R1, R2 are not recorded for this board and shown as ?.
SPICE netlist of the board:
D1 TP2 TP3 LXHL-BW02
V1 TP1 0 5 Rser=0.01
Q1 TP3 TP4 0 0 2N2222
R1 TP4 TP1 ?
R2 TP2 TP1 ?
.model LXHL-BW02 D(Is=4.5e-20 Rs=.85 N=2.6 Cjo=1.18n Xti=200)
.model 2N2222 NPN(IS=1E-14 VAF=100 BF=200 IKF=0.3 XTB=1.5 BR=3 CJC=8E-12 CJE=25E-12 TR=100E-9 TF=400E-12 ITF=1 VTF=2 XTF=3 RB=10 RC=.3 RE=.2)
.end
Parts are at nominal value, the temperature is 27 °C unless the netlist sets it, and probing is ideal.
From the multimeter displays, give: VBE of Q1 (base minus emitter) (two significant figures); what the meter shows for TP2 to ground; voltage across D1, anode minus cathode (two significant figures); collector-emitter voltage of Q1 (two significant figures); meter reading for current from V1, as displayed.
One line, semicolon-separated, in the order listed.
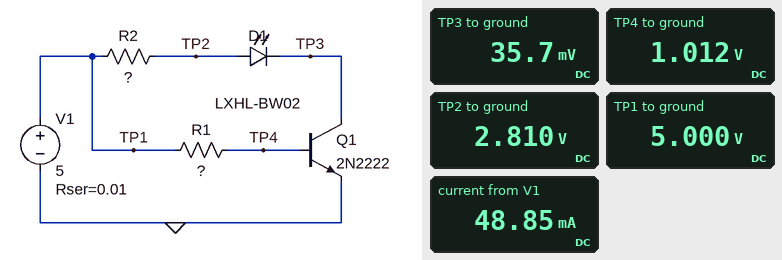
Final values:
1.0 V; 2.810 V; 2.8 V; 36 mV; 48.85 mA
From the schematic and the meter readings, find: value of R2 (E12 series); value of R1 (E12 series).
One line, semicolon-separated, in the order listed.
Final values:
82 Ω; 180 Ω
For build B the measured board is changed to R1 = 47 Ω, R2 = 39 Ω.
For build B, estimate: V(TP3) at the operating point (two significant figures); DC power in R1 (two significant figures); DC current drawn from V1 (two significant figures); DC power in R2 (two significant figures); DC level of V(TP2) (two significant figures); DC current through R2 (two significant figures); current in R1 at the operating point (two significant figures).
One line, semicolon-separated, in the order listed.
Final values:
60 mV; 250 mW; 130 mA; 110 mW; 2.9 V; 54 mA; 73 mA
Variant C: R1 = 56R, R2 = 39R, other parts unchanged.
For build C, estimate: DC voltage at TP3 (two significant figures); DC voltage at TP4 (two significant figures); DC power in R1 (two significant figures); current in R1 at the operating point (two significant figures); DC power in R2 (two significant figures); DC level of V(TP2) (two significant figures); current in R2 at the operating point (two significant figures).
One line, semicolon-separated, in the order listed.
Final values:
59 mV; 1.5 V; 220 mW; 63 mA; 110 mW; 2.9 V; 54 mA
